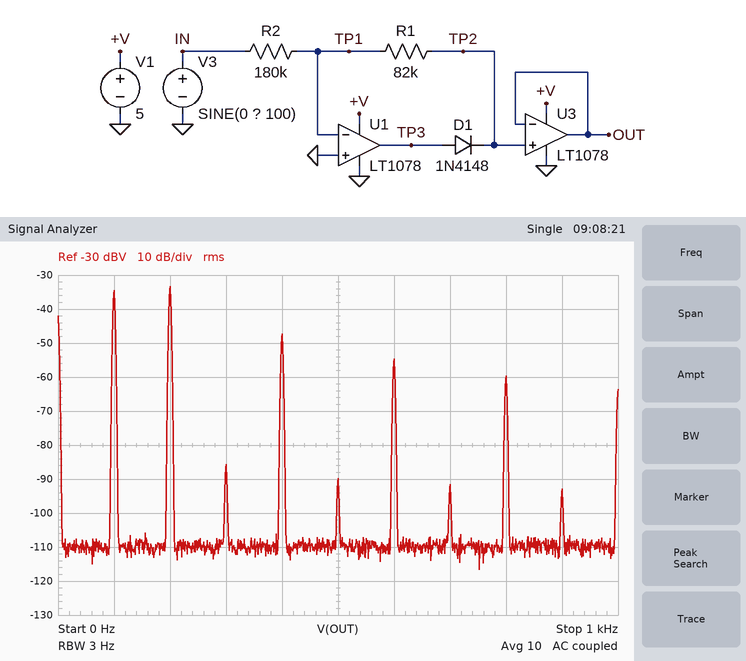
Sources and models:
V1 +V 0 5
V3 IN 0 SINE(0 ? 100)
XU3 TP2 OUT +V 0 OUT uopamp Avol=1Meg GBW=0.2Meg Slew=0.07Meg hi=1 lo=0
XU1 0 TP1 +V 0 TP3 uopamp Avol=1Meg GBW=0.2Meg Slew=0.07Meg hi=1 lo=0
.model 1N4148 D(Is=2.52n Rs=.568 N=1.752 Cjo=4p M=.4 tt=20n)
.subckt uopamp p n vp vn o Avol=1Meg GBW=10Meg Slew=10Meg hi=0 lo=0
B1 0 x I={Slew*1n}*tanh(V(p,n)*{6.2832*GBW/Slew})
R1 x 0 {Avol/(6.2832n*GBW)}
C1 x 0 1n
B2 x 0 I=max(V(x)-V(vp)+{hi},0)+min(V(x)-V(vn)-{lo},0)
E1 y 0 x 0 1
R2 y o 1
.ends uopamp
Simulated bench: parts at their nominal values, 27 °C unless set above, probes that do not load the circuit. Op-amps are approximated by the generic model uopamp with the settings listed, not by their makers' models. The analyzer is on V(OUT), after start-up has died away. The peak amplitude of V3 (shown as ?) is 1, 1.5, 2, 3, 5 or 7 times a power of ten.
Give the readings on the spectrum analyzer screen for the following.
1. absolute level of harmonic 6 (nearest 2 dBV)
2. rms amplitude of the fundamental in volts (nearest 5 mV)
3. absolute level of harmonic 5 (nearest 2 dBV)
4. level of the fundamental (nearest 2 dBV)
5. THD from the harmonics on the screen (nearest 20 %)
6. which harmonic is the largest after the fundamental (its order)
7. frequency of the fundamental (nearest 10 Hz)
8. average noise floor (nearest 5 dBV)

-54 dBV
20 mV
-90 dBV
-34 dBV
120 %
2
100 Hz
-110 dBV
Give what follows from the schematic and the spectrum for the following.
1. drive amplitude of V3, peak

100 mV
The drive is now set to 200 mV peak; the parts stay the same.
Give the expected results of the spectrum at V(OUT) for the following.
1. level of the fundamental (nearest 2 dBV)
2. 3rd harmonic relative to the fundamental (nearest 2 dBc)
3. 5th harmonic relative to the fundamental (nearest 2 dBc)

-28 dBV
-54 dBc
-58 dBc
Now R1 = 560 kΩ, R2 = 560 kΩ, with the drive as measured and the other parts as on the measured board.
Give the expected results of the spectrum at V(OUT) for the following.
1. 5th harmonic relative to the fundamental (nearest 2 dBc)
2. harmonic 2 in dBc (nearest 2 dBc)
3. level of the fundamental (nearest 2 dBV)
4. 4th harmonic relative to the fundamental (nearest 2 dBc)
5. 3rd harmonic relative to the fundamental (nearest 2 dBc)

-26 dBc
30 dBc
-60 dBV
16 dBc
-16 dBc
